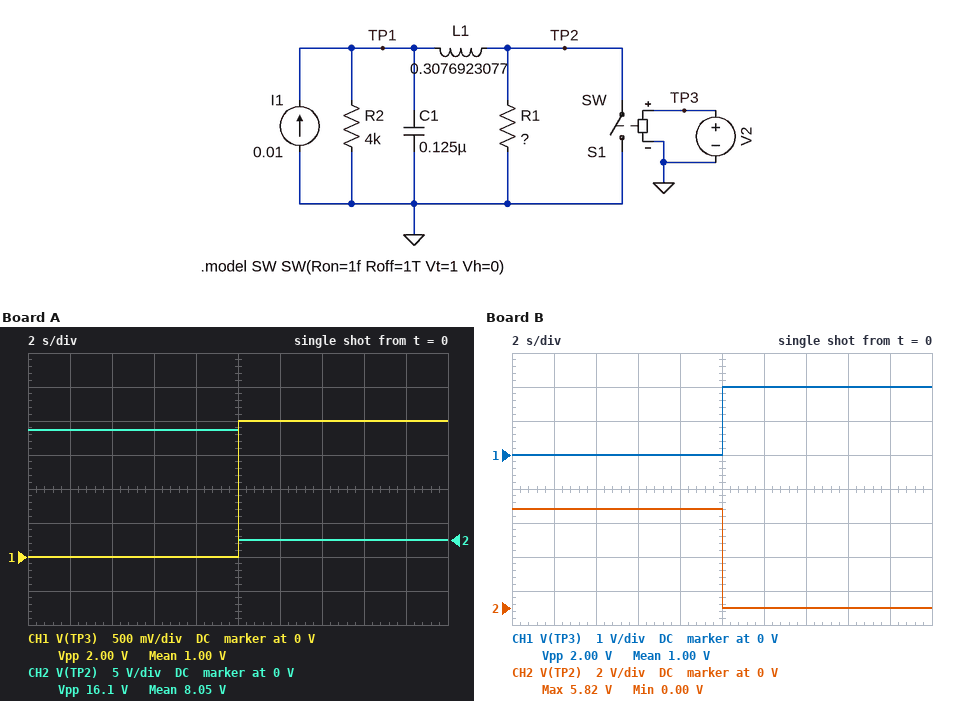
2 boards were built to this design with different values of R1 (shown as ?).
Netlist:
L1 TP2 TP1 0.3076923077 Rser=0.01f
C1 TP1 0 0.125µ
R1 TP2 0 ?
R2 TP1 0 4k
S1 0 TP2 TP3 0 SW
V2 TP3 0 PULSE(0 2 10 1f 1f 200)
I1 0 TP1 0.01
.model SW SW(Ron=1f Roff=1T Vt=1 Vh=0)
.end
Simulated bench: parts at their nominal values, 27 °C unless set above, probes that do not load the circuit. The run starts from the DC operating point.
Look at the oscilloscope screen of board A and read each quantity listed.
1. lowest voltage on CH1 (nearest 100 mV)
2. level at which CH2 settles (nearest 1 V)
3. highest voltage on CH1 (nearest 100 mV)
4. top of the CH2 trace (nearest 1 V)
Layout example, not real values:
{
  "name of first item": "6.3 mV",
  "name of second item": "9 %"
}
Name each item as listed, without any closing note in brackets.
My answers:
{
  "lowest voltage on CH1": "0 V",
  "level at which CH2 settles": "0 V",
  "highest voltage on CH1": "2.0 V",
  "top of the CH2 trace": "16 V"
}
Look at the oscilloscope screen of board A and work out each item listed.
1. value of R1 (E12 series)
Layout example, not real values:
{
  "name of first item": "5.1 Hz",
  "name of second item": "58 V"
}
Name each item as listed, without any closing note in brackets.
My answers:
{
  "value of R1": "2.7 kΩ"
}
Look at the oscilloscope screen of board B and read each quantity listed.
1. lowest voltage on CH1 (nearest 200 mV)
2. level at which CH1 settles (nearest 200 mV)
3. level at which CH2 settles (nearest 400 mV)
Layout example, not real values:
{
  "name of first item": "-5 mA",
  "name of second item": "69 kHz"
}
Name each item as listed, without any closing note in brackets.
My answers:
{
  "lowest voltage on CH1": "0 V",
  "level at which CH1 settles": "2.0 V",
  "level at which CH2 settles": "0 V"
}
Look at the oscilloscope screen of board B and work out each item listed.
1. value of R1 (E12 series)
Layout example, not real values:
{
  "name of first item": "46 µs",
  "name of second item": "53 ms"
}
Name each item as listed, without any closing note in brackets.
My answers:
{
  "value of R1": "680 Ω"
}
